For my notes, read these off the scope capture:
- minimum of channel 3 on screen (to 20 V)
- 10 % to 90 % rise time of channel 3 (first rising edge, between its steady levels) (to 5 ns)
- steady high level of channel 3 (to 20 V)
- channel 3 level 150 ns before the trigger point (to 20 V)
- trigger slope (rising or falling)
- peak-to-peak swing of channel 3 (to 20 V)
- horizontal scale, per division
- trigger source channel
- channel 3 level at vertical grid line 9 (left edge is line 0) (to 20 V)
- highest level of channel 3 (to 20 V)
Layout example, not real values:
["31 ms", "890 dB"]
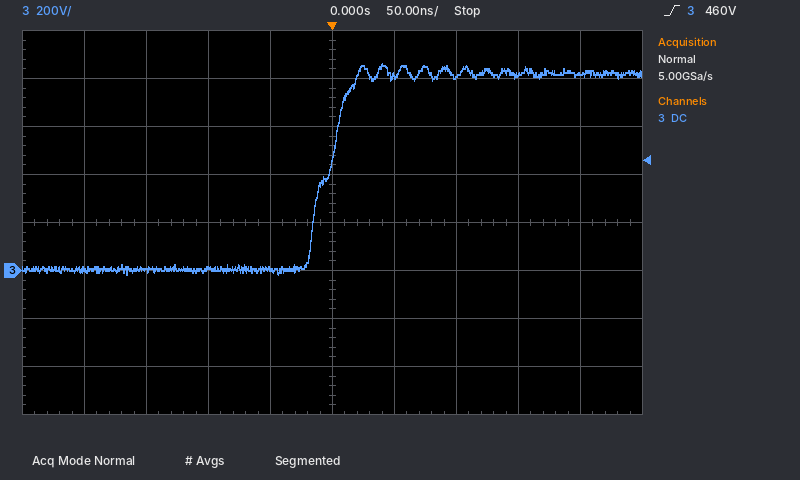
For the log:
["-20 V", "30 ns", "820 V", "0 V", "rising", "880 V", "50 ns", "channel 3", "820 V", "860 V"]
